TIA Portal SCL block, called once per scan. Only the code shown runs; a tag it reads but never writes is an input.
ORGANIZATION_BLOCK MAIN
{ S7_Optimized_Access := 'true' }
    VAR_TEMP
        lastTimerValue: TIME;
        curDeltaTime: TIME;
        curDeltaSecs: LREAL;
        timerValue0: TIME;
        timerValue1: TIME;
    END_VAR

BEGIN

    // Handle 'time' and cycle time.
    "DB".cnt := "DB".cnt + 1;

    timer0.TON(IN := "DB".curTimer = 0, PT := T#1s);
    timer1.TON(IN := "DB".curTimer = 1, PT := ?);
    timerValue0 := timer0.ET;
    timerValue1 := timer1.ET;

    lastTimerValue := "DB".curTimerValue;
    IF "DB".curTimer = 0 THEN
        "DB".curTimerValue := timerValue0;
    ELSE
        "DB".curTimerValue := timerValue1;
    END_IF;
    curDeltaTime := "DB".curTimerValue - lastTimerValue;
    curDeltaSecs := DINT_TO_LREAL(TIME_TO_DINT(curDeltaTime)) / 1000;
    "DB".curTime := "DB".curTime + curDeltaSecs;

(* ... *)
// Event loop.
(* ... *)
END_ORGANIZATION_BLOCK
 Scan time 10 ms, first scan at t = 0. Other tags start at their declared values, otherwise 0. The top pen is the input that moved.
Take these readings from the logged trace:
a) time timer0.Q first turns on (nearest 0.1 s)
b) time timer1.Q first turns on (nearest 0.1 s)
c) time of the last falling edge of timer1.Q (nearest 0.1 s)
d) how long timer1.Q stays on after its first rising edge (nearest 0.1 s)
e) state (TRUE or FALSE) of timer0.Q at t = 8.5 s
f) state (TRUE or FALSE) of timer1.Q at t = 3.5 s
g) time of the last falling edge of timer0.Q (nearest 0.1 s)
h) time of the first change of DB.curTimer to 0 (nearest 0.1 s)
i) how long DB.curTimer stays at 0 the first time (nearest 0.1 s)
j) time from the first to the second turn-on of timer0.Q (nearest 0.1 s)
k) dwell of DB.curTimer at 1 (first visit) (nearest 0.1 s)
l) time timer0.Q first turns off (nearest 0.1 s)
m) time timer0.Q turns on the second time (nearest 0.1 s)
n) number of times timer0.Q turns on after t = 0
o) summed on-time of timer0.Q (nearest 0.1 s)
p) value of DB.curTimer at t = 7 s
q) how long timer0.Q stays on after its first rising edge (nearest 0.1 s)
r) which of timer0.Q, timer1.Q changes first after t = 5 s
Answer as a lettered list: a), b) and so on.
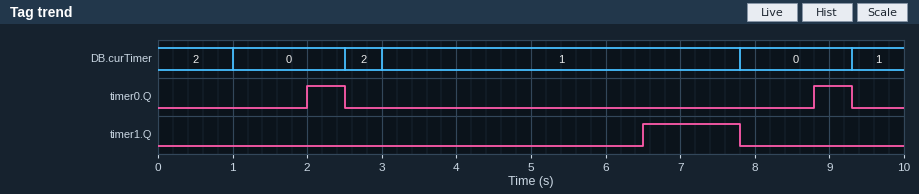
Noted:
a) 2.0 s
b) 6.5 s
c) 7.8 s
d) 1.3 s
e) FALSE
f) FALSE
g) 9.3 s
h) 1.0 s
i) 1.5 s
j) 6.8 s
k) 4.8 s
l) 2.5 s
m) 8.8 s
n) 2
o) 1.0 s
p) 1
q) 0.5 s
r) timer1.Q
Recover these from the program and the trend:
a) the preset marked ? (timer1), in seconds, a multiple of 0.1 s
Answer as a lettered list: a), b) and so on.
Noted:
a) 3.5 s
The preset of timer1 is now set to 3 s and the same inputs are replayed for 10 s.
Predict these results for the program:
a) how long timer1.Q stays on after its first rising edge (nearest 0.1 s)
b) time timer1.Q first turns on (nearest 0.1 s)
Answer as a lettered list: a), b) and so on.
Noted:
a) 1.8 s
b) 6.0 s
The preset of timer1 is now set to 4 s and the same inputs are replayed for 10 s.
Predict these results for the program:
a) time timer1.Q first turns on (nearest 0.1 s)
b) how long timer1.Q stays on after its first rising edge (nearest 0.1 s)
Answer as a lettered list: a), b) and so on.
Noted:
a) 7.0 s
b) 0.8 s
